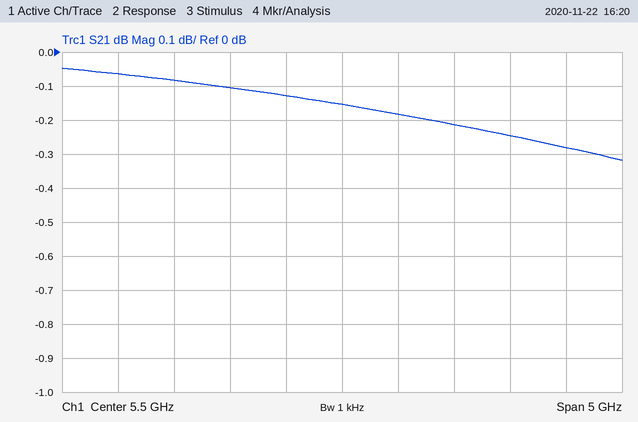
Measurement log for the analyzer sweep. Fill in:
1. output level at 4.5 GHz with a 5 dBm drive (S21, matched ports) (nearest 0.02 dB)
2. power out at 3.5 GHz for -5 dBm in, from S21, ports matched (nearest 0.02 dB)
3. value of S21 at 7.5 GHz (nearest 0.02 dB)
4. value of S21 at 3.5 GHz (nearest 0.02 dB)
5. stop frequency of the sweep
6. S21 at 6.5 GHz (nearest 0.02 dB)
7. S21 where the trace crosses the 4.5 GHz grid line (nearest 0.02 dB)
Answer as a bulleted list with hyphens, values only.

- 4.90 dBm
- -5.06 dBm
- -0.28 dB
- -0.06 dB
- 8 GHz
- -0.22 dB
- -0.10 dB
